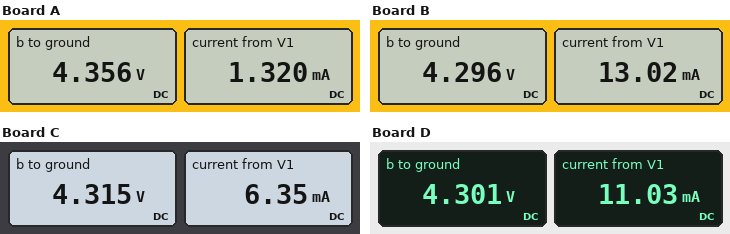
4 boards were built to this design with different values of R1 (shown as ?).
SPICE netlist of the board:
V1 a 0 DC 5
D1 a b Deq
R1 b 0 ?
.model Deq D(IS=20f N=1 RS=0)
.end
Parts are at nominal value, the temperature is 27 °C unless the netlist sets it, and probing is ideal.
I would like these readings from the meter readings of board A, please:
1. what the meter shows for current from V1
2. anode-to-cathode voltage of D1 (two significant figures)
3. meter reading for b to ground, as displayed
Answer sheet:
1.320 mA
640 mV
4.356 V
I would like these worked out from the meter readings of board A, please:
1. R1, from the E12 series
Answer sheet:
3.3 kΩ
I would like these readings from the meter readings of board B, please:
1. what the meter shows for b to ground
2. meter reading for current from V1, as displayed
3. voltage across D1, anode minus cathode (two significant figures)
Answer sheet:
4.296 V
13.02 mA
700 mV
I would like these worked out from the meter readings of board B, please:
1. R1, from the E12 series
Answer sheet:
330 Ω
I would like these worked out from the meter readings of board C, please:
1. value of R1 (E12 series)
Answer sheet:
680 Ω
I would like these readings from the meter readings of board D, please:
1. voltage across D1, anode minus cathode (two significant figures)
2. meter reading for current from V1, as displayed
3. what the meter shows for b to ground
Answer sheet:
700 mV
11.03 mA
4.301 V
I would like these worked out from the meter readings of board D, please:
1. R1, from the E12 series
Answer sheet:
390 Ω
